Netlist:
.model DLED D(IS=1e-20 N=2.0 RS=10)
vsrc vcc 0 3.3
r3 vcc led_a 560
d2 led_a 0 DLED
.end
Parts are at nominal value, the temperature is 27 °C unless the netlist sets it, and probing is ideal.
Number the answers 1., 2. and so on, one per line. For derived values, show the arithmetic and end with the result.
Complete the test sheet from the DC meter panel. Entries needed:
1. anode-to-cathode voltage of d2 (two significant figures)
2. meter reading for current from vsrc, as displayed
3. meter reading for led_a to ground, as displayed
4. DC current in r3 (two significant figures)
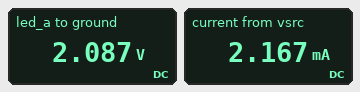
1. 2.087 V = 2.1 V
2. 2.167 mA
3. 2.087 V
4. (3.3 V - 2.087 V) / 560 Ω = 2.2 mA
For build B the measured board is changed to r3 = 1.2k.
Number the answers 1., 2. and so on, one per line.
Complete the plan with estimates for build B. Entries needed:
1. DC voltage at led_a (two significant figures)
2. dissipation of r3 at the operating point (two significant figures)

1. 2.0 V
2. 1.3 mW
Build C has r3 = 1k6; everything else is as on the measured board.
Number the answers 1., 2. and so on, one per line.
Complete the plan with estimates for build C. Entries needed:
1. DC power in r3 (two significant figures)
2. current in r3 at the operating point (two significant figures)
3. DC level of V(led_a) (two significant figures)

1. 1.0 mW
2. 800 µA
3. 2.0 V
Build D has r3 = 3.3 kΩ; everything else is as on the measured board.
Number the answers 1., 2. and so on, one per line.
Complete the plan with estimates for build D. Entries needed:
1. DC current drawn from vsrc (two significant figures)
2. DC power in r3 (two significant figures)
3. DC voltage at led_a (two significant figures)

1. 400 µA
2. 530 µW
3. 2.0 V
